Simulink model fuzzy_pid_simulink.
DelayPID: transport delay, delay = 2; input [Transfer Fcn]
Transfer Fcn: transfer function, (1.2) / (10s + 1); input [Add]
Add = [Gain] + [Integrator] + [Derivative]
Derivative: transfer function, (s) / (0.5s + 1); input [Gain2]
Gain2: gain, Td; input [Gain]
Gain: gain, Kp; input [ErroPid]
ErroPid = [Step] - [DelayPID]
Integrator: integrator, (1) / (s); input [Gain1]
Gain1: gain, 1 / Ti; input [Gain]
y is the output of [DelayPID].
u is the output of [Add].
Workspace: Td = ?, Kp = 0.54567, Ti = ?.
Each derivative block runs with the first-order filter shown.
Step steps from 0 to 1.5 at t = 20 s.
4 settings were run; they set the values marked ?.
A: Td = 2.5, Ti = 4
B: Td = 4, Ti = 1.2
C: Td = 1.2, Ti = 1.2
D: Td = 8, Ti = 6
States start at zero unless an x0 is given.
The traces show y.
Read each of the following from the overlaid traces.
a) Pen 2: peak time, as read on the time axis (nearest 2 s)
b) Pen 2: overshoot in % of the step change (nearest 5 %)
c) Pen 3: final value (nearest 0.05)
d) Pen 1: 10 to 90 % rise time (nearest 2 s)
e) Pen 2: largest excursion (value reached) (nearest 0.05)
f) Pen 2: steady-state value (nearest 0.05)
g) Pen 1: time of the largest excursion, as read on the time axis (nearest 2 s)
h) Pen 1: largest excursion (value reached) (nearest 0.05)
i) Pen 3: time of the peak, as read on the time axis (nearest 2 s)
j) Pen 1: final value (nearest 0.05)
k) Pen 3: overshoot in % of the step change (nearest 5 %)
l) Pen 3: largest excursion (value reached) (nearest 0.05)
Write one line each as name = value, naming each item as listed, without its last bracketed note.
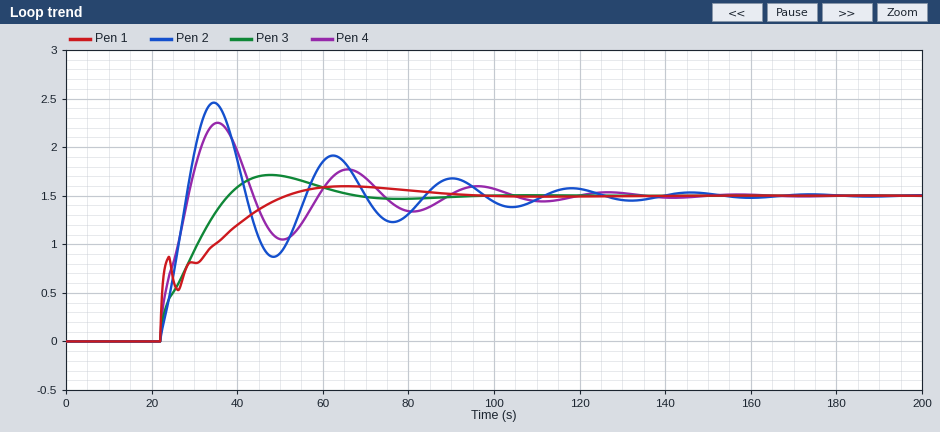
Pen 2: peak time, as read on the time axis = 34 s
Pen 2: overshoot in % of the step change = 65 %
Pen 3: final value = 1.50
Pen 1: 10 to 90 % rise time = 22 s
Pen 2: largest excursion (value reached) = 2.45
Pen 2: steady-state value = 1.50
Pen 1: time of the largest excursion, as read on the time axis = 66 s
Pen 1: largest excursion (value reached) = 1.60
Pen 3: time of the peak, as read on the time axis = 48 s
Pen 1: final value = 1.50
Pen 3: overshoot in % of the step change = 15 %
Pen 3: largest excursion (value reached) = 1.70
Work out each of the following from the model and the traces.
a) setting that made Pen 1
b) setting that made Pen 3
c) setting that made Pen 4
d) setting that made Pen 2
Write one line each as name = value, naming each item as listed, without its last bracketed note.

setting that made Pen 1 = D
setting that made Pen 3 = A
setting that made Pen 4 = B
setting that made Pen 2 = C
